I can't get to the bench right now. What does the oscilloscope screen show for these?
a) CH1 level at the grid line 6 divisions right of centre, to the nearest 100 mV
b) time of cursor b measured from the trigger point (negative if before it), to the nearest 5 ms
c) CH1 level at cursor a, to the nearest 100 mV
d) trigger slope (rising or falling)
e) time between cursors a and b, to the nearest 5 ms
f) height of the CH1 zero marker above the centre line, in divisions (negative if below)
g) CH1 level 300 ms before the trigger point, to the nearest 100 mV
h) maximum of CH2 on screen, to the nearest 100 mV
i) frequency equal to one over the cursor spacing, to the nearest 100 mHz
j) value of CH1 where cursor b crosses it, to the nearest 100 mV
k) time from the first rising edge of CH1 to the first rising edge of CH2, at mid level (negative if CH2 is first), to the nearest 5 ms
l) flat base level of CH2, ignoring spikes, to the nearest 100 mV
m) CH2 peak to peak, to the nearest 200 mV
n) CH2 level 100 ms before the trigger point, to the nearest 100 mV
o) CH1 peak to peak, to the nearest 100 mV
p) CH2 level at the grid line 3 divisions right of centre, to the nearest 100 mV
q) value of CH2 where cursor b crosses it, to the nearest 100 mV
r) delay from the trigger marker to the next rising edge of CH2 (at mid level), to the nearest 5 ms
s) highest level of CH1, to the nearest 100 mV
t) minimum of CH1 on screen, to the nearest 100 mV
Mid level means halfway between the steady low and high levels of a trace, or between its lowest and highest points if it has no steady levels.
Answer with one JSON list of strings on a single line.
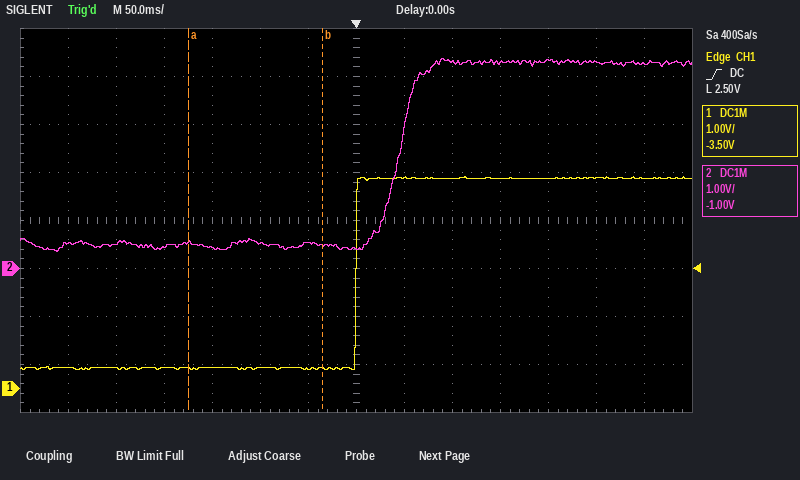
["4.4 V", "-35 ms", "400 mV", "rising", "140 ms", "-3.5 div", "400 mV", "4.4 V", "7.1 Hz", "400 mV", "+45 ms", "500 mV", "4.0 V", "500 mV", "4.0 V", "4.3 V", "500 mV", "45 ms", "4.4 V", "400 mV"]
